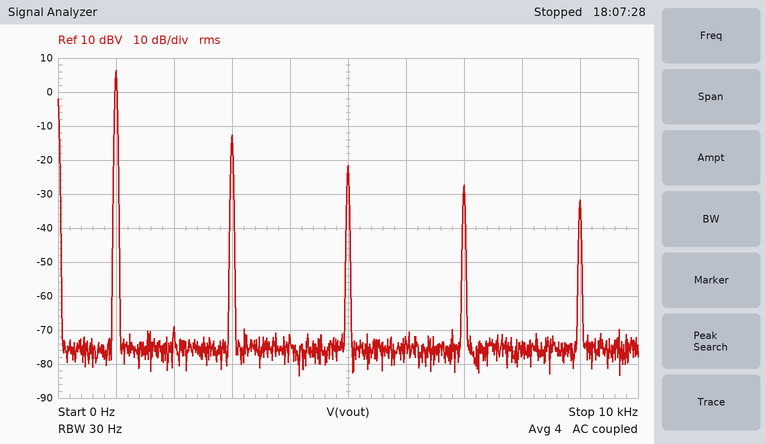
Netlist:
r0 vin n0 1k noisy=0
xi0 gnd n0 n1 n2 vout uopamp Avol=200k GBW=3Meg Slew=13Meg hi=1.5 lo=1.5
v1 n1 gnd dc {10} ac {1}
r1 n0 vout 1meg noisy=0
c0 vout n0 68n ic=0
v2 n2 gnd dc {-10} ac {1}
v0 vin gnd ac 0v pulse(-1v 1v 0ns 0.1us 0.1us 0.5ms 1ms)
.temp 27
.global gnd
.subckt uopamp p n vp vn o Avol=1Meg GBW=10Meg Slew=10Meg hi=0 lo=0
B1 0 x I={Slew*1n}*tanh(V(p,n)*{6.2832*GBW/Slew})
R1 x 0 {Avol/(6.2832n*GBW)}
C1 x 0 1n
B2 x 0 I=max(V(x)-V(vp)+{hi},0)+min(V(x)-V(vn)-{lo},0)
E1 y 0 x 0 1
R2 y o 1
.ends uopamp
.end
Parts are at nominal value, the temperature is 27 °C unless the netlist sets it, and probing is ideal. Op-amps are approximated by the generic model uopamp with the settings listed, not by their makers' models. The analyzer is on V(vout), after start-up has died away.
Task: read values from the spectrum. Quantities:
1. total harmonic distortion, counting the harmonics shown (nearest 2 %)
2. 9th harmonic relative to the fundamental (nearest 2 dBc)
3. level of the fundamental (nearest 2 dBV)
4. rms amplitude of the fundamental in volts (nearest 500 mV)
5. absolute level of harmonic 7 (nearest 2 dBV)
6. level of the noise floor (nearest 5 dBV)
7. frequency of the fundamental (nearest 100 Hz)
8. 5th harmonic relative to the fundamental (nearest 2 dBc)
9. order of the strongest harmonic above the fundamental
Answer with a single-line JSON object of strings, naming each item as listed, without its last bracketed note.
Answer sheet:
{"total harmonic distortion, counting the harmonics shown": "12 %", "9th harmonic relative to the fundamental": "-38 dBc", "level of the fundamental": "6 dBV", "rms amplitude of the fundamental in volts": "2.0 V", "absolute level of harmonic 7": "-28 dBV", "level of the noise floor": "-75 dBV", "frequency of the fundamental": "1.0 kHz", "5th harmonic relative to the fundamental": "-28 dBc", "order of the strongest harmonic above the fundamental": "3"}
